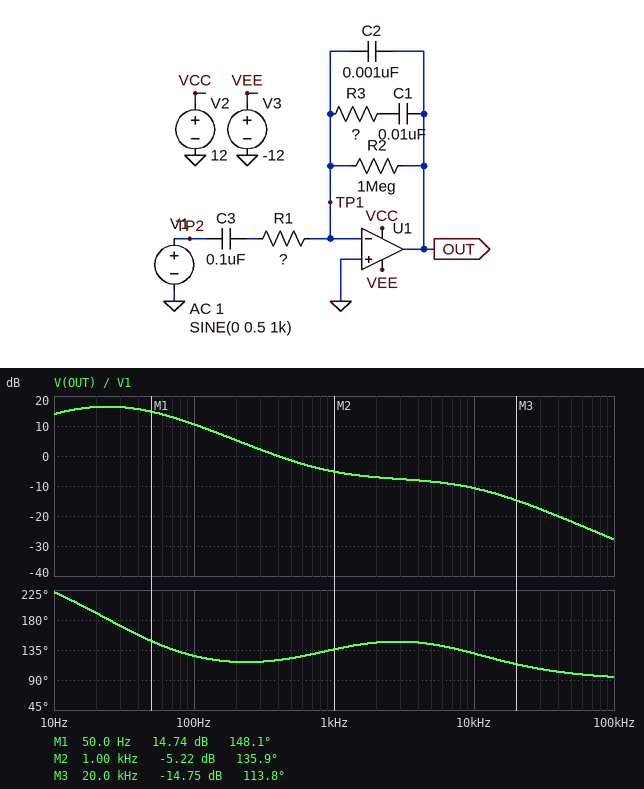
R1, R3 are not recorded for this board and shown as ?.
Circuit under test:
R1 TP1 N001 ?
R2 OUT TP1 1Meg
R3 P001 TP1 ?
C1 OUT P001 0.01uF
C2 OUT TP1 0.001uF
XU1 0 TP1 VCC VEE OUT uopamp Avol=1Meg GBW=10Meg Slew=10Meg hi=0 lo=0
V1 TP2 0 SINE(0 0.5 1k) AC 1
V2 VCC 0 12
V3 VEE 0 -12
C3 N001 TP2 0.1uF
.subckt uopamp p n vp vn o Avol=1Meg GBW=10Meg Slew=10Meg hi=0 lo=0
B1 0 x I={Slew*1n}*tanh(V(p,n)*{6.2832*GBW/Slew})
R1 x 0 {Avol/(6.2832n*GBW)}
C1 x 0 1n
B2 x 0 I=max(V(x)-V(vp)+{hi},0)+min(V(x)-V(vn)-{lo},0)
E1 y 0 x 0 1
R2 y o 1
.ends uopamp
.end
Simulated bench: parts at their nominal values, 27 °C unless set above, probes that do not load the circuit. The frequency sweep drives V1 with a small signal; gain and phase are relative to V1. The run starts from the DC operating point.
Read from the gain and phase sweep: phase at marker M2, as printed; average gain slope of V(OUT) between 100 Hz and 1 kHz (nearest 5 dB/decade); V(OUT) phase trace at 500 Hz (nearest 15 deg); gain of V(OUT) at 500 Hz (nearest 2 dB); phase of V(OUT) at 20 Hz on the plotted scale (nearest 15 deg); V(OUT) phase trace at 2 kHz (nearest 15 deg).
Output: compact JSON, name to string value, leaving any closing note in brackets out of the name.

{"phase at marker M2, as printed": "135.9 deg", "average gain slope of V(OUT) between 100 Hz and 1 kHz": "-15 dB/decade", "V(OUT) phase trace at 500 Hz": "120 deg", "gain of V(OUT) at 500 Hz": "-2 dB", "phase of V(OUT) at 20 Hz on the plotted scale": "195 deg", "V(OUT) phase trace at 2 kHz": "150 deg"}
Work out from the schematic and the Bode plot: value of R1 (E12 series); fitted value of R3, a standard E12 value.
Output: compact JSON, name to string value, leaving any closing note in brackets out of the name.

{"value of R1": "39 kΩ", "fitted value of R3, a standard E12 value": "18 kΩ"}
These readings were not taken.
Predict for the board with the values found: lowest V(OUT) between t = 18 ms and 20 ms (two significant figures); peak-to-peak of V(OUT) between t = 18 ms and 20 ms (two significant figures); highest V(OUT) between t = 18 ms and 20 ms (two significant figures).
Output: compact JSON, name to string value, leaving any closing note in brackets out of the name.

{"lowest V(OUT) between t = 18 ms and 20 ms": "-260 mV", "peak-to-peak of V(OUT) between t = 18 ms and 20 ms": "550 mV", "highest V(OUT) between t = 18 ms and 20 ms": "290 mV"}
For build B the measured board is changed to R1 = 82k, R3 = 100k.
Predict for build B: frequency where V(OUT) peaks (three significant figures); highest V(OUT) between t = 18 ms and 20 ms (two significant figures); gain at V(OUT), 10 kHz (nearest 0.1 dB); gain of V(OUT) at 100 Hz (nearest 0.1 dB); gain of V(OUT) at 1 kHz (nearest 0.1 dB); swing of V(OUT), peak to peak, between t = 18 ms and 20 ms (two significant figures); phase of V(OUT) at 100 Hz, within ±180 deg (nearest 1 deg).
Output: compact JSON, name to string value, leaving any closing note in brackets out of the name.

{"frequency where V(OUT) peaks": "16.3 Hz", "highest V(OUT) between t = 18 ms and 20 ms": "470 mV", "gain at V(OUT), 10 kHz": "-14.4 dB", "gain of V(OUT) at 100 Hz": "5.4 dB", "gain of V(OUT) at 1 kHz": "-0.8 dB", "swing of V(OUT), peak to peak, between t = 18 ms and 20 ms": "920 mV", "phase of V(OUT) at 100 Hz, within ±180 deg": "138 deg"}
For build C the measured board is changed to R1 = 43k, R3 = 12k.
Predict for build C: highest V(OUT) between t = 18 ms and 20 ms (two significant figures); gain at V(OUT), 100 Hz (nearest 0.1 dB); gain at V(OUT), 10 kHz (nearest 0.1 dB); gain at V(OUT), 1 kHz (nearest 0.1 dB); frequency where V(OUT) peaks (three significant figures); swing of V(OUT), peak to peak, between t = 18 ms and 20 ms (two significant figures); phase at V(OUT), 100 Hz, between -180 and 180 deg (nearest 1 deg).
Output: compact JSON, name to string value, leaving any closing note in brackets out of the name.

{"highest V(OUT) between t = 18 ms and 20 ms": "220 mV", "gain at V(OUT), 100 Hz": "9.8 dB", "gain at V(OUT), 10 kHz": "-13.6 dB", "gain at V(OUT), 1 kHz": "-7.6 dB", "frequency where V(OUT) peaks": "23.0 Hz", "swing of V(OUT), peak to peak, between t = 18 ms and 20 ms": "420 mV", "phase at V(OUT), 100 Hz, between -180 and 180 deg": "122 deg"}
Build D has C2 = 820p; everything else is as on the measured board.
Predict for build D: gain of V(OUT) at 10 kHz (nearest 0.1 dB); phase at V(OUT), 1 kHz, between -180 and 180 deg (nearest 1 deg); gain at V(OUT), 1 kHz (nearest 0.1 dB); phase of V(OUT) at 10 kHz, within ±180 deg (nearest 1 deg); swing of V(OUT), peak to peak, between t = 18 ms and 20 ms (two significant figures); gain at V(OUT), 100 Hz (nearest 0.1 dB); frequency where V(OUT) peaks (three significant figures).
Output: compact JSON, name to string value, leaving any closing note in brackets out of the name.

{"gain of V(OUT) at 10 kHz": "-9.8 dB", "phase at V(OUT), 1 kHz, between -180 and 180 deg": "137 deg", "gain at V(OUT), 1 kHz": "-5.1 dB", "phase of V(OUT) at 10 kHz, within ±180 deg": "135 deg", "swing of V(OUT), peak to peak, between t = 18 ms and 20 ms": "560 mV", "gain at V(OUT), 100 Hz": "10.7 dB", "frequency where V(OUT) peaks": "24.3 Hz"}
